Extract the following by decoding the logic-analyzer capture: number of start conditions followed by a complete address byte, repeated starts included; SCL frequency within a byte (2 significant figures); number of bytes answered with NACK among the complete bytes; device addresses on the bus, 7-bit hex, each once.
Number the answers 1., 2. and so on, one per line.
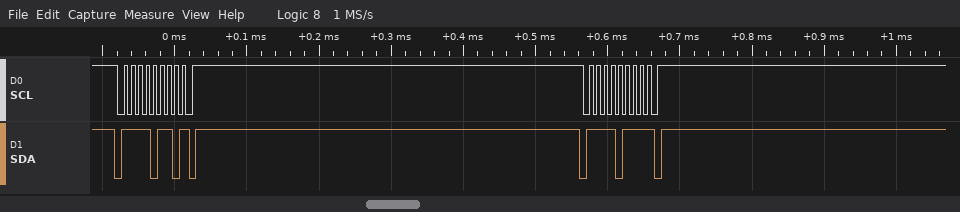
1. 2
2. 100 kHz
3. 2
4. 0x7B
